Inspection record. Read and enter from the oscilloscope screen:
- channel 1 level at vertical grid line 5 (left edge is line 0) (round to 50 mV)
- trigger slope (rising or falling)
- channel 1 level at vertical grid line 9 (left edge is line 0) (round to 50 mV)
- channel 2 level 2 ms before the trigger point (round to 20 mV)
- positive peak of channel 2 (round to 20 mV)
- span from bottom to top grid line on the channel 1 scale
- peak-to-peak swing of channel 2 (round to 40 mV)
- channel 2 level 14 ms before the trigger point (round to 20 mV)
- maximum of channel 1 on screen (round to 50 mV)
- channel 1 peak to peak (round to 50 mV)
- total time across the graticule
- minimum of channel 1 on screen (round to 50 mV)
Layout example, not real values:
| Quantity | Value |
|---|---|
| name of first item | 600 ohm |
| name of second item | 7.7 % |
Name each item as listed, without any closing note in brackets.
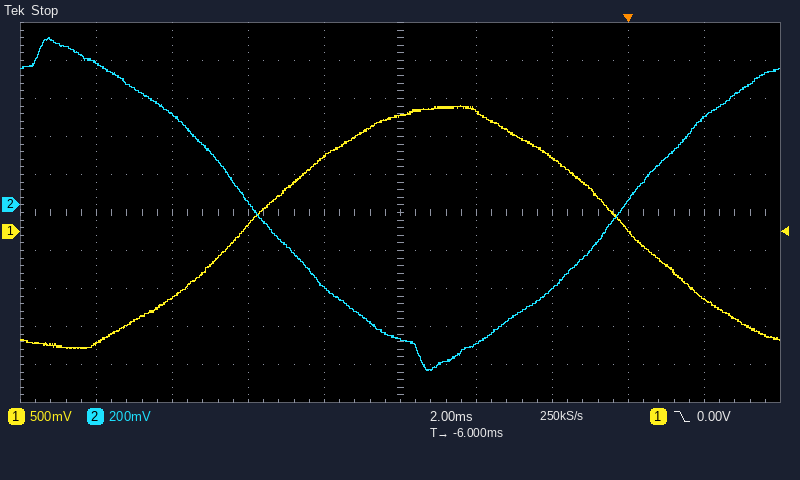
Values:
| Quantity | Value |
|---|---|
| channel 1 level at vertical grid line 5 (left edge is line 0) | 1.50 V |
| trigger slope | falling |
| channel 1 level at vertical grid line 9 (left edge is line 0) | -900 mV |
| channel 2 level 2 ms before the trigger point | -440 mV |
| positive peak of channel 2 | 880 mV |
| span from bottom to top grid line on the channel 1 scale | 5 V |
| peak-to-peak swing of channel 2 | 1.76 V |
| channel 2 level 14 ms before the trigger point | 740 mV |
| maximum of channel 1 on screen | 1.65 V |
| channel 1 peak to peak | 3.20 V |
| total time across the graticule | 20 ms |
| minimum of channel 1 on screen | -1.55 V |
